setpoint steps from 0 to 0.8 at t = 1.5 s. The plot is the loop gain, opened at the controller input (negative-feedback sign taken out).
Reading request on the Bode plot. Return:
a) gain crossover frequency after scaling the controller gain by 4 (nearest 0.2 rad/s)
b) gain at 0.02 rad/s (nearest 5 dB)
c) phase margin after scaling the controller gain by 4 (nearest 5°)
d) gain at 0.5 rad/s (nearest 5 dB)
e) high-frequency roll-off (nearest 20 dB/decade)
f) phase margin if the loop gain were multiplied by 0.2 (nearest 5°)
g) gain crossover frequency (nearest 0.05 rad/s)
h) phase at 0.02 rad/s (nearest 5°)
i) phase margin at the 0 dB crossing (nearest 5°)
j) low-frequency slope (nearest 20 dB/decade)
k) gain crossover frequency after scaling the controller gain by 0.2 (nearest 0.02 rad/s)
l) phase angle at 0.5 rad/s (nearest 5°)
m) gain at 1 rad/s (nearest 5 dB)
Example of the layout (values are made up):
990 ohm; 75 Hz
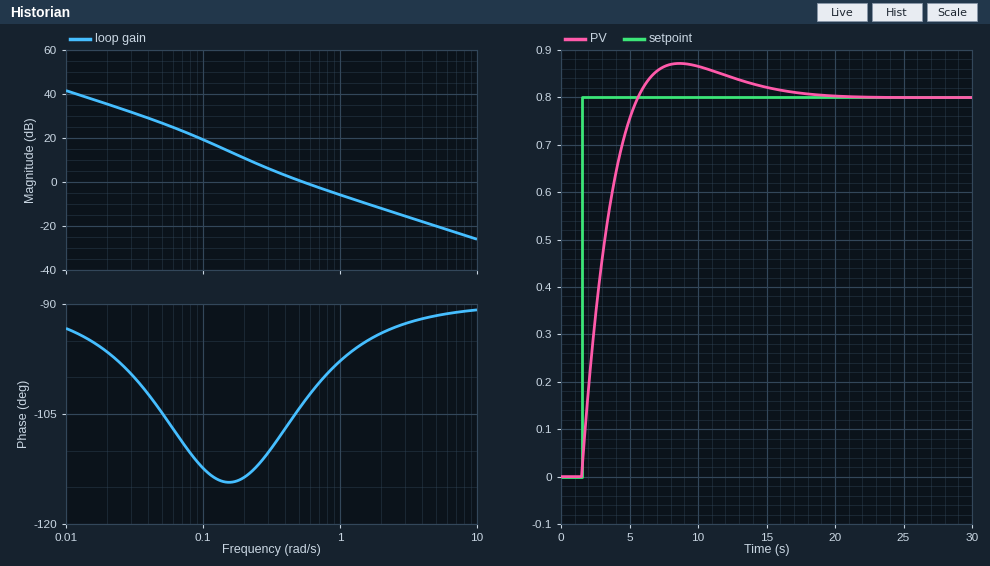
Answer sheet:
2.0 rad/s; 35 dB; 85°; 0 dB; -20 dB/decade; 65°; 0.55 rad/s; -95°; 75°; -20 dB/decade; 0.16 rad/s; -105°; -5 dB
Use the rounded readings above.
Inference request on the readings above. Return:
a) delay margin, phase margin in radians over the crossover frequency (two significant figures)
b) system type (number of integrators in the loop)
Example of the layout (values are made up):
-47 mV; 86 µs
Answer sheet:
2.4 s; 1
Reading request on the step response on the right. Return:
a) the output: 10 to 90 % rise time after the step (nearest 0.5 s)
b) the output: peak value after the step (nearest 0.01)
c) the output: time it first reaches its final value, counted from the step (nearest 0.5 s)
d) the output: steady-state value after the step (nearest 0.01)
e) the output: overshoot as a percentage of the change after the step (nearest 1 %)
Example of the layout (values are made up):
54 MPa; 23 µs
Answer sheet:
3.0 s; 0.87; 4.0 s; 0.80; 9 %
